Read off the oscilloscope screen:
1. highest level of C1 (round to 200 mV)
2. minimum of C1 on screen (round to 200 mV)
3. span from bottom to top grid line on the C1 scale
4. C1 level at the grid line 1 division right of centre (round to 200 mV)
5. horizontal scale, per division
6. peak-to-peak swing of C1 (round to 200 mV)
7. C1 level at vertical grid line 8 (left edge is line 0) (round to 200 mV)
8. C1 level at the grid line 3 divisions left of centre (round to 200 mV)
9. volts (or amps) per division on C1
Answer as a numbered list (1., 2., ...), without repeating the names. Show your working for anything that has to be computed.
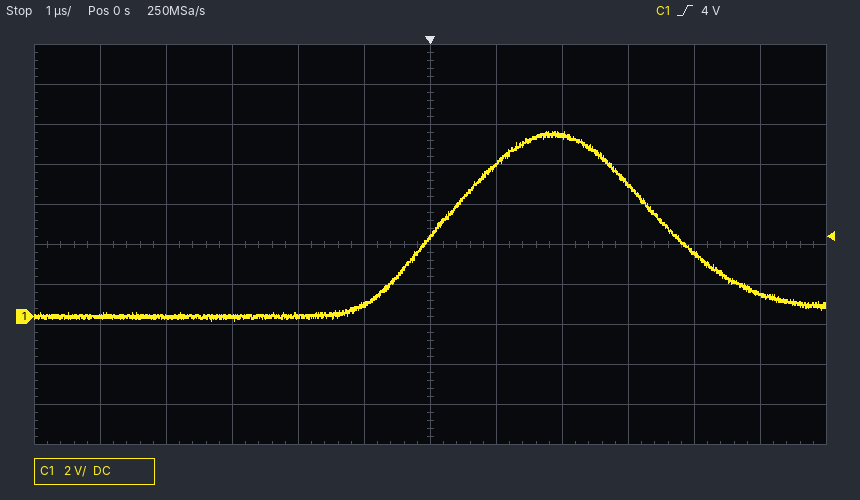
1. 9.2 V
2. -200 mV
3. 20 V
4. 7.6 V
5. 1 µs
6. 9.2 V − (-200 mV) = 9.4 V
7. 9.0 V
8. 0.0 V
9. 2 V
